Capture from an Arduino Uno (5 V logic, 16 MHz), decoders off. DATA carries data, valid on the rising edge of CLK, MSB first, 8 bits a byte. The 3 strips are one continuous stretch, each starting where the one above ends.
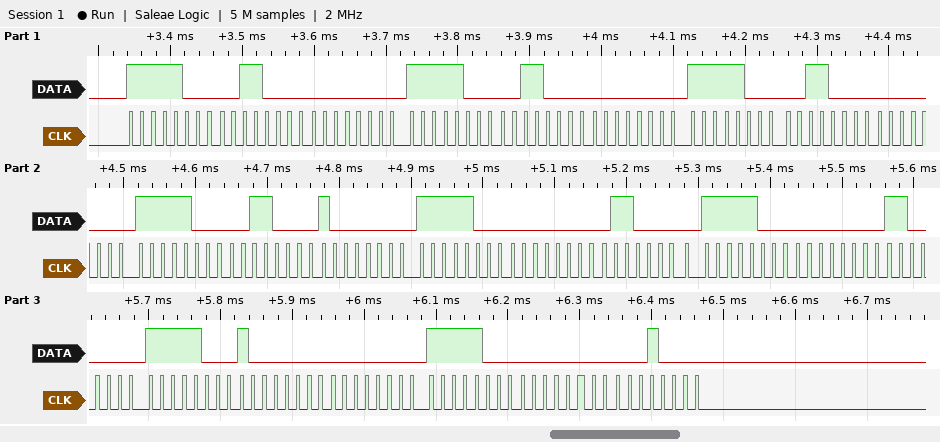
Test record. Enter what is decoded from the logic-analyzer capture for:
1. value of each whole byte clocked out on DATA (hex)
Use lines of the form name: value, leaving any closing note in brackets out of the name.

value of each whole byte clocked out on DATA: F8 30 00 F8 30 00 F8 30 00 F8 30 80 F8 00 60 F8 00 C0 F8 80 00 F8 00 10
